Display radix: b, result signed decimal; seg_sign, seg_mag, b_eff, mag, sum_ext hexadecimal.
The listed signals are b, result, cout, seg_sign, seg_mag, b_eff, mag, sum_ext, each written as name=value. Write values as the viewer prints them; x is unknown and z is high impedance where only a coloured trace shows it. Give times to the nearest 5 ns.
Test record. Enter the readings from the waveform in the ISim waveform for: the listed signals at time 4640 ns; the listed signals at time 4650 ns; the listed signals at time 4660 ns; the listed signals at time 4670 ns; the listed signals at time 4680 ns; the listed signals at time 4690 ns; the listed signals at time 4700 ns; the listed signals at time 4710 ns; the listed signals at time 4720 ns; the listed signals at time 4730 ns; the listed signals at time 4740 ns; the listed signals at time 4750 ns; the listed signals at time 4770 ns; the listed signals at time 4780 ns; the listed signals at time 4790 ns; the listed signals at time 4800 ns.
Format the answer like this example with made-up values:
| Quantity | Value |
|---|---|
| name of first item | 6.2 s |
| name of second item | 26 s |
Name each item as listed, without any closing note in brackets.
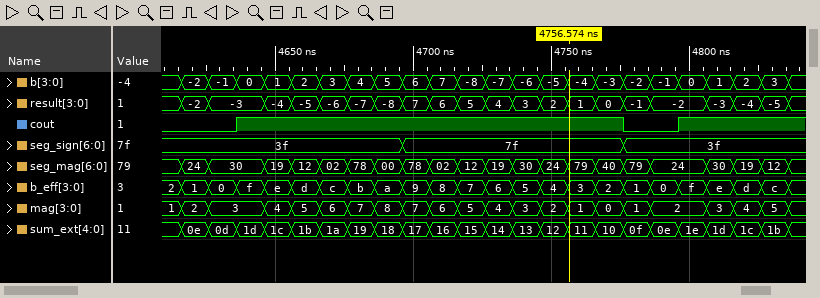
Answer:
| Quantity | Value |
|---|---|
| the listed signals at time 4640 ns | b=0, result=-3, cout=1, seg_sign=3f, seg_mag=30, b_eff=f, mag=3, sum_ext=1d |
| the listed signals at time 4650 ns | b=1, result=-4, cout=1, seg_sign=3f, seg_mag=19, b_eff=e, mag=4, sum_ext=1c |
| the listed signals at time 4660 ns | b=2, result=-5, cout=1, seg_sign=3f, seg_mag=12, b_eff=d, mag=5, sum_ext=1b |
| the listed signals at time 4670 ns | b=3, result=-6, cout=1, seg_sign=3f, seg_mag=02, b_eff=c, mag=6, sum_ext=1a |
| the listed signals at time 4680 ns | b=4, result=-7, cout=1, seg_sign=3f, seg_mag=78, b_eff=b, mag=7, sum_ext=19 |
| the listed signals at time 4690 ns | b=5, result=-8, cout=1, seg_sign=3f, seg_mag=00, b_eff=a, mag=8, sum_ext=18 |
| the listed signals at time 4700 ns | b=6, result=7, cout=1, seg_sign=7f, seg_mag=78, b_eff=9, mag=7, sum_ext=17 |
| the listed signals at time 4710 ns | b=7, result=6, cout=1, seg_sign=7f, seg_mag=02, b_eff=8, mag=6, sum_ext=16 |
| the listed signals at time 4720 ns | b=-8, result=5, cout=1, seg_sign=7f, seg_mag=12, b_eff=7, mag=5, sum_ext=15 |
| the listed signals at time 4730 ns | b=-7, result=4, cout=1, seg_sign=7f, seg_mag=19, b_eff=6, mag=4, sum_ext=14 |
| the listed signals at time 4740 ns | b=-6, result=3, cout=1, seg_sign=7f, seg_mag=30, b_eff=5, mag=3, sum_ext=13 |
| the listed signals at time 4750 ns | b=-5, result=2, cout=1, seg_sign=7f, seg_mag=24, b_eff=4, mag=2, sum_ext=12 |
| the listed signals at time 4770 ns | b=-3, result=0, cout=1, seg_sign=7f, seg_mag=40, b_eff=2, mag=0, sum_ext=10 |
| the listed signals at time 4780 ns | b=-2, result=-1, cout=0, seg_sign=3f, seg_mag=79, b_eff=1, mag=1, sum_ext=0f |
| the listed signals at time 4790 ns | b=-1, result=-2, cout=0, seg_sign=3f, seg_mag=24, b_eff=0, mag=2, sum_ext=0e |
| the listed signals at time 4800 ns | b=0, result=-2, cout=1, seg_sign=3f, seg_mag=24, b_eff=f, mag=2, sum_ext=1e |
